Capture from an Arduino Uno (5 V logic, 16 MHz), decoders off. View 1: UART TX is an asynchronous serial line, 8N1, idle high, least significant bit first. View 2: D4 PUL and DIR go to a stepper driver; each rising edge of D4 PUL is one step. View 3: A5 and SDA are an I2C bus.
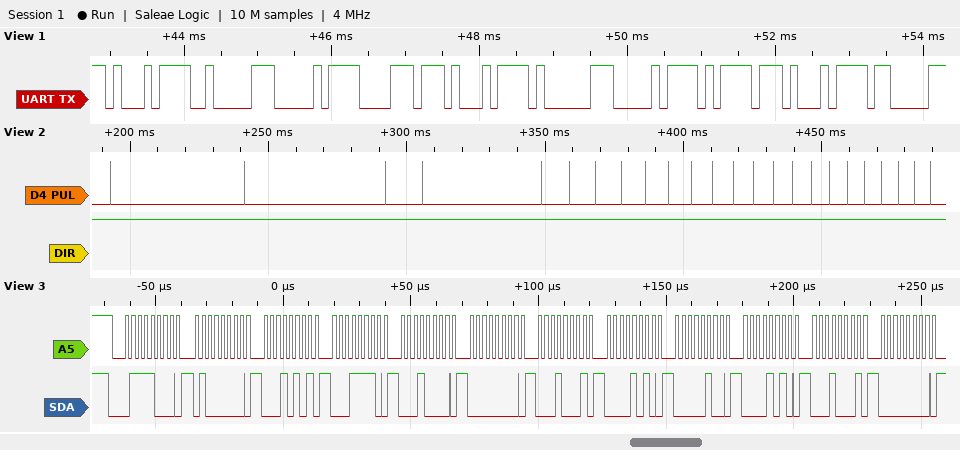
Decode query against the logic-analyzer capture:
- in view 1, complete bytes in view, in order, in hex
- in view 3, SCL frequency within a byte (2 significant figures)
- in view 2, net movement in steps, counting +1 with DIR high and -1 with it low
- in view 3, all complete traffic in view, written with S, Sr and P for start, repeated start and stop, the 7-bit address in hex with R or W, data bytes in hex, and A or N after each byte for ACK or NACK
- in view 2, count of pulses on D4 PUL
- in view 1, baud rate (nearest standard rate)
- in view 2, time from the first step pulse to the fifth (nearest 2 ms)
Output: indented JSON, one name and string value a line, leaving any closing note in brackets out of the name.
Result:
{
  "in view 1, complete bytes in view, in order, in hex": "D1 82 D0 B8 D1 81 D0 BD D1 83",
  "in view 3, SCL frequency within a byte": "400 kHz",
  "in view 2, net movement in steps, counting +1 with DIR high and -1 with it low": "+24",
  "in view 3, all complete traffic in view, written with S, Sr and P for start, repeated start and stop, the 7-bit address in hex with R or W, data bytes in hex, and A or N after each byte for ACK or NACK": "S 3CW A 40 A 15 A 1E A 10 A 00 A 11 A 0A A 04 A 0A A 11 A 00 A",
  "in view 2, count of pulses on D4 PUL": "24",
  "in view 1, baud rate": "9600 baud",
  "in view 2, time from the first step pulse to the fifth": "156 ms"
}
